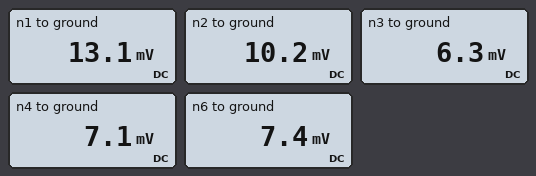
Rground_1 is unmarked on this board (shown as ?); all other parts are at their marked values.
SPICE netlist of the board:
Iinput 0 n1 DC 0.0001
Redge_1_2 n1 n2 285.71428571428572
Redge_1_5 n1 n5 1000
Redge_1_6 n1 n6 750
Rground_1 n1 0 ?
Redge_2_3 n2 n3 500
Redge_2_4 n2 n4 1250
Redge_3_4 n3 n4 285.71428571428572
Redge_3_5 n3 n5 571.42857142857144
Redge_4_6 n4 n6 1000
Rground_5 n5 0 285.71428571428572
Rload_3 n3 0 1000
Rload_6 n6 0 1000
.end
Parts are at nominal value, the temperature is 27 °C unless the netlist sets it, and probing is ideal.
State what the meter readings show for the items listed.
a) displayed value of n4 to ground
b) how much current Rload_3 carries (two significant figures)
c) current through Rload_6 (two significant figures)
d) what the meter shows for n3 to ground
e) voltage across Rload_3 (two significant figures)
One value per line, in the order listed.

7.1 mV
6.3 µA
7.4 µA
6.3 mV
6.3 mV
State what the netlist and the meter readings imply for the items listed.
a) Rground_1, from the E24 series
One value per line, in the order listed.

180 Ω
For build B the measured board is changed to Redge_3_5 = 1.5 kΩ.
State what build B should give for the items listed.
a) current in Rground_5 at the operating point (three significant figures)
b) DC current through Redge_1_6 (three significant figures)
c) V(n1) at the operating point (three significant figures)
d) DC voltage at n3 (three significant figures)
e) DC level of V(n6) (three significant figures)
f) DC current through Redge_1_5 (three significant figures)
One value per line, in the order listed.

12.1 µA
7.51 µA
13.2 mV
6.98 mV
7.57 mV
9.75 µA
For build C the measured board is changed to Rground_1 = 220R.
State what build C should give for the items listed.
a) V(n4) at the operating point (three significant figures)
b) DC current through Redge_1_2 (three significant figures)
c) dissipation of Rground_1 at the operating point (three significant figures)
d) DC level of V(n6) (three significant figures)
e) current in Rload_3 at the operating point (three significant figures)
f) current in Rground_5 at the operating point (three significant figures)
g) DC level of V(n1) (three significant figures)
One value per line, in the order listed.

8.16 mV
11.8 µA
1.04 µW
8.49 mV
7.25 µA
15.6 µA
15.1 mV
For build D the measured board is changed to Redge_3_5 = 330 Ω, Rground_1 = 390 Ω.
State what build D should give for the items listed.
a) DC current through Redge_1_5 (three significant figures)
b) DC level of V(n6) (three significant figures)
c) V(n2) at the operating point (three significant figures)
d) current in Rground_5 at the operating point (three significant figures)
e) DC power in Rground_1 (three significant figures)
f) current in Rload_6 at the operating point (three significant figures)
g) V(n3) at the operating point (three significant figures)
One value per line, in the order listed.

14.7 µA
11.9 mV
16.4 mV
23.5 µA
1.18 µW
11.9 µA
9.64 mV
